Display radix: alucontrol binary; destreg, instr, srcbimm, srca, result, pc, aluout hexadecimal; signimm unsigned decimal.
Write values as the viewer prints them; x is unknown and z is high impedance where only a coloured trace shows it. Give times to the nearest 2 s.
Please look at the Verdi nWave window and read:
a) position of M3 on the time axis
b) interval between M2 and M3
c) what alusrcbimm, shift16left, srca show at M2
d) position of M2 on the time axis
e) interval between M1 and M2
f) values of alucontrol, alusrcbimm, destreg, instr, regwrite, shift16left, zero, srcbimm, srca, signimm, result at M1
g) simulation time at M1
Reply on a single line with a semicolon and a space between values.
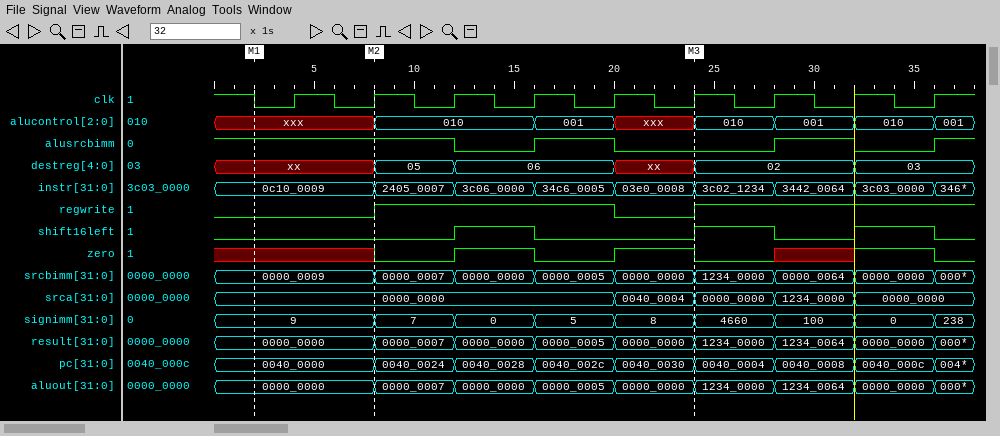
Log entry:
24 s; 16 s; alusrcbimm=1, shift16left=0, srca=0000_0000; 8 s; 6 s; alucontrol=xxx, alusrcbimm=1, destreg=xx, instr=0c10_0009, regwrite=0, shift16left=0, zero=x, srcbimm=0000_0009, srca=0000_0000, signimm=9, result=0000_0000; 2 s
